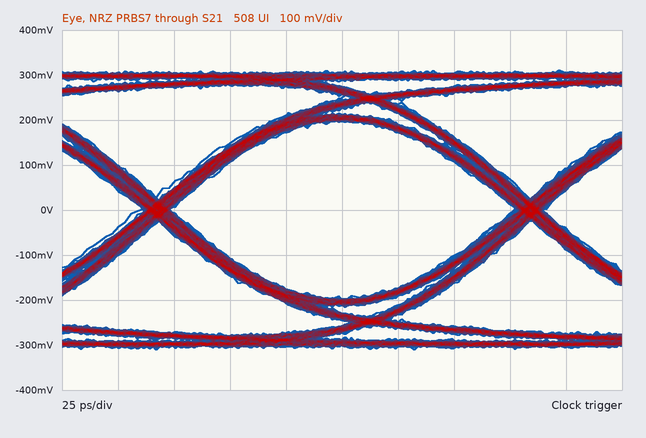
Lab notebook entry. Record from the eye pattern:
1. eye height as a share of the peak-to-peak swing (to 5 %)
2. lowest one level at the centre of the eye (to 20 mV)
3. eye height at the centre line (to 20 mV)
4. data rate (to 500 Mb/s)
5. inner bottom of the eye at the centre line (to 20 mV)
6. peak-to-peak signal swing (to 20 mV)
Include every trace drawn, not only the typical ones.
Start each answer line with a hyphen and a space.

- 65 %
- 200 mV
- 400 mV
- 6.0 Gb/s
- -200 mV
- 620 mV
